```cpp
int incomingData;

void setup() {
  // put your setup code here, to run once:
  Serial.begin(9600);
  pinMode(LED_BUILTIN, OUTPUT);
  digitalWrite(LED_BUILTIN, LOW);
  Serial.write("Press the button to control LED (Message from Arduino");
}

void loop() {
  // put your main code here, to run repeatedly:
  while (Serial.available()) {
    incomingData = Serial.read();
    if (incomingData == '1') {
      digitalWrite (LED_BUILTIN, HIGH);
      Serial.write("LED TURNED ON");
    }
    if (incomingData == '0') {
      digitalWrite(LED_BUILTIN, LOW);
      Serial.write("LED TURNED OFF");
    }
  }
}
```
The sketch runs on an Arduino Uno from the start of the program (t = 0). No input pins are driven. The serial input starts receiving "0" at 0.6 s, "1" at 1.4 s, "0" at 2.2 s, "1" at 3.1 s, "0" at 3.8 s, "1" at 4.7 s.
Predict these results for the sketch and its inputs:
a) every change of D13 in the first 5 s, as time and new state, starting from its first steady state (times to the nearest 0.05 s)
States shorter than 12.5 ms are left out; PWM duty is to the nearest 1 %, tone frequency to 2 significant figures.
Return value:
0 s low; 1.4 s high; 2.2 s low; 3.1 s high; 3.8 s low; 4.7 s high
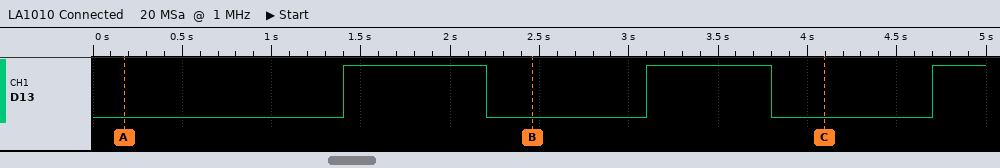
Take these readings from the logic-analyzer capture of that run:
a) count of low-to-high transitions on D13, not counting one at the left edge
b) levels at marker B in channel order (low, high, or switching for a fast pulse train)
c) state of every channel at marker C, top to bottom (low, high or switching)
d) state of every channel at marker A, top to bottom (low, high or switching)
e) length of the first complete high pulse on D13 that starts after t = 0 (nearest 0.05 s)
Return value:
3
D13 low
D13 low
D13 low
0.80 s
